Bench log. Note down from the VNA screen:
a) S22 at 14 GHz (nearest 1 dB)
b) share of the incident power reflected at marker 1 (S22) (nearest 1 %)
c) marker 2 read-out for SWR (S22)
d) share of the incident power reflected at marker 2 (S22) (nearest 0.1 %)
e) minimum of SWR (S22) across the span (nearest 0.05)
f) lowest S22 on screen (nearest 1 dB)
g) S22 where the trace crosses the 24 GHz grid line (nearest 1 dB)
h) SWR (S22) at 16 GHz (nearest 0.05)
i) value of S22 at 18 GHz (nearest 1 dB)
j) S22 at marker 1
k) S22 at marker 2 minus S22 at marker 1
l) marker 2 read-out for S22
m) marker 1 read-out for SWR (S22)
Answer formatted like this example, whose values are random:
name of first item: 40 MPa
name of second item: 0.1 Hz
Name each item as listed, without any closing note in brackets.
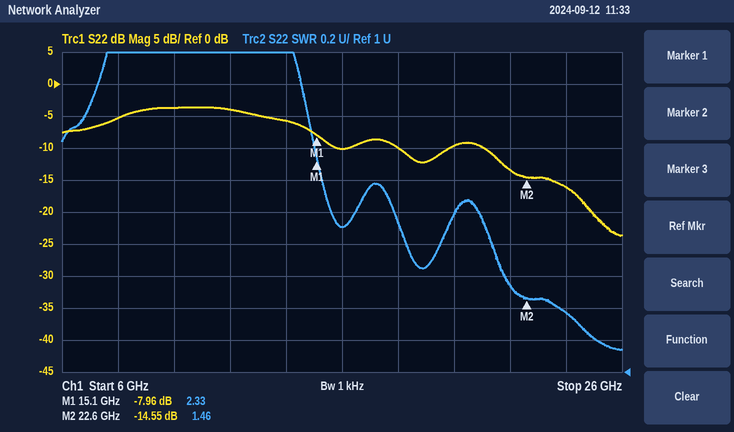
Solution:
S22 at 14 GHz: -6 dB
share of the incident power reflected at marker 1 (S22): 16 %
marker 2 read-out for SWR: 1.46
share of the incident power reflected at marker 2 (S22): 3.5 %
minimum of SWR (S22) across the span: 1.15
lowest S22 on screen: -24 dB
S22 where the trace crosses the 24 GHz grid line: -16 dB
SWR (S22) at 16 GHz: 1.90
value of S22 at 18 GHz: -10 dB
S22 at marker 1: -7.96 dB
S22 at marker 2 minus S22 at marker 1: -6.59 dB
marker 2 read-out for S22: -14.55 dB
marker 1 read-out for SWR: 2.33
